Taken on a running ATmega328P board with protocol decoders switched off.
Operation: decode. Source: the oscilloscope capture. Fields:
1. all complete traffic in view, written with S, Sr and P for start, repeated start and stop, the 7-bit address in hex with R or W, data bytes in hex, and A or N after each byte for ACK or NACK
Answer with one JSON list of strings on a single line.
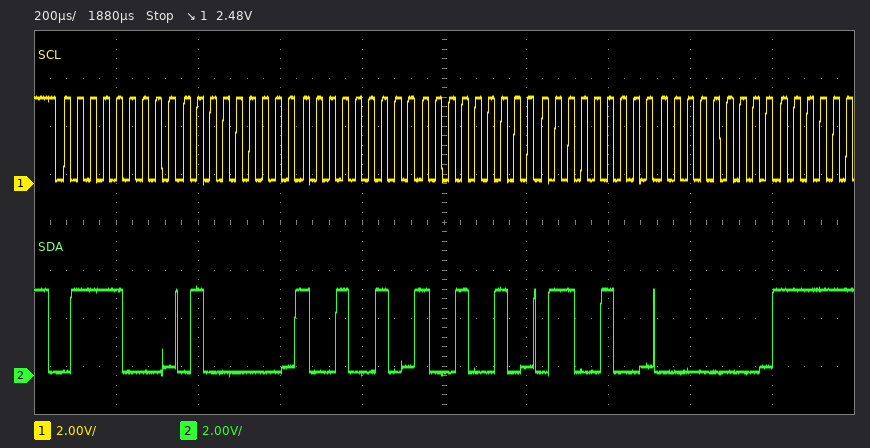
["S 3CW A 40 A 92 A 92 A 64 A 00 A"]
